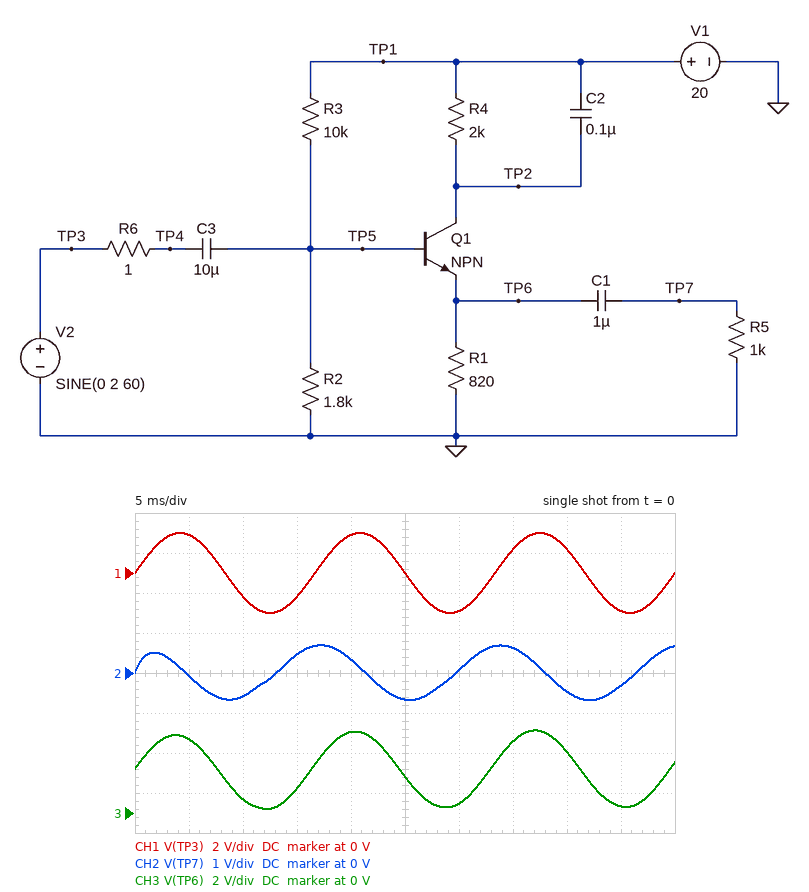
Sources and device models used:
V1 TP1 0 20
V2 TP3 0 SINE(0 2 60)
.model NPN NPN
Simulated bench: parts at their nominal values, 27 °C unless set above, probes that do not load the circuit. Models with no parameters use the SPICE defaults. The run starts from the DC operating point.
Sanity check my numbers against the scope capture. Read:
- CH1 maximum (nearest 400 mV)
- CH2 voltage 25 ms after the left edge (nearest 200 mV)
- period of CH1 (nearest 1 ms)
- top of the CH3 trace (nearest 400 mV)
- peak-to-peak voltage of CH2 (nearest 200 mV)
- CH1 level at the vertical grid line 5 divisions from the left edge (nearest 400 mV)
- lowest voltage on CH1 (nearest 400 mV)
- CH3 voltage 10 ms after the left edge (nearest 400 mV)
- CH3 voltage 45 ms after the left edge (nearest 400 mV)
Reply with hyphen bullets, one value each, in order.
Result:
- 2.0 V
- -600 mV
- 17 ms
- 4.0 V
- 1.4 V
- 0 V
- -2.0 V
- 800 mV
- 400 mV
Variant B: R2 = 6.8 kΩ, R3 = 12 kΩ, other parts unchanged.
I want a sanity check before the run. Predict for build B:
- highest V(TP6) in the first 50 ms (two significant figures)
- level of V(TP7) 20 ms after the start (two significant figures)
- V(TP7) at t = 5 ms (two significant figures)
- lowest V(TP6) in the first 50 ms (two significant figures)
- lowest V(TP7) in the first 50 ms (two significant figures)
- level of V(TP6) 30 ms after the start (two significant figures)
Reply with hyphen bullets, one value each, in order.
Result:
- 7.1 V
- 270 mV
- -170 mV
- 2.8 V
- -680 mV
- 3.0 V
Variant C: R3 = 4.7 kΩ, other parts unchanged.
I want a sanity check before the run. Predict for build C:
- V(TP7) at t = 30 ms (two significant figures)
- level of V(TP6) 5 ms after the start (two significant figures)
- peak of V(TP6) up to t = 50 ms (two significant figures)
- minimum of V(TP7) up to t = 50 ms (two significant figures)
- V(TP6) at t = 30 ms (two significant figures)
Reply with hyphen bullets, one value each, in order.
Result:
- 120 mV
- 5.9 V
- 6.3 V
- -660 mV
- 2.8 V
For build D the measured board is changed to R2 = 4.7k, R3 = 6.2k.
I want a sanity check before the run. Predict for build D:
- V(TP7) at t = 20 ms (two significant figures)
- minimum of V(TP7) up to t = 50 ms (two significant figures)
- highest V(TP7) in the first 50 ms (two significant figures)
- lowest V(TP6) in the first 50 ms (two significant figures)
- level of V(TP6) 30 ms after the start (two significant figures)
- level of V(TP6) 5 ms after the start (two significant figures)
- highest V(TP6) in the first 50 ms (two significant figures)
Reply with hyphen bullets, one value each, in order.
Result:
- 200 mV
- -620 mV
- 700 mV
- 3.6 V
- 3.9 V
- 7.0 V
- 7.4 V
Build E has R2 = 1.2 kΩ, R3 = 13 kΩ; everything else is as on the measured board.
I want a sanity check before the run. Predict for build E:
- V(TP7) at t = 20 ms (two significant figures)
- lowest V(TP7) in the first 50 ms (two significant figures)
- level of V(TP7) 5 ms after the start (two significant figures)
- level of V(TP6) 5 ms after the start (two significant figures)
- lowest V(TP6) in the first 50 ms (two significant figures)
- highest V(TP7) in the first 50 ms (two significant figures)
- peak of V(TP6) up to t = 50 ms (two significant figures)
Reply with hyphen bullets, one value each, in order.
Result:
- 290 mV
- -630 mV
- -100 mV
- 2.2 V
- 13 mV
- 630 mV
- 2.8 V
